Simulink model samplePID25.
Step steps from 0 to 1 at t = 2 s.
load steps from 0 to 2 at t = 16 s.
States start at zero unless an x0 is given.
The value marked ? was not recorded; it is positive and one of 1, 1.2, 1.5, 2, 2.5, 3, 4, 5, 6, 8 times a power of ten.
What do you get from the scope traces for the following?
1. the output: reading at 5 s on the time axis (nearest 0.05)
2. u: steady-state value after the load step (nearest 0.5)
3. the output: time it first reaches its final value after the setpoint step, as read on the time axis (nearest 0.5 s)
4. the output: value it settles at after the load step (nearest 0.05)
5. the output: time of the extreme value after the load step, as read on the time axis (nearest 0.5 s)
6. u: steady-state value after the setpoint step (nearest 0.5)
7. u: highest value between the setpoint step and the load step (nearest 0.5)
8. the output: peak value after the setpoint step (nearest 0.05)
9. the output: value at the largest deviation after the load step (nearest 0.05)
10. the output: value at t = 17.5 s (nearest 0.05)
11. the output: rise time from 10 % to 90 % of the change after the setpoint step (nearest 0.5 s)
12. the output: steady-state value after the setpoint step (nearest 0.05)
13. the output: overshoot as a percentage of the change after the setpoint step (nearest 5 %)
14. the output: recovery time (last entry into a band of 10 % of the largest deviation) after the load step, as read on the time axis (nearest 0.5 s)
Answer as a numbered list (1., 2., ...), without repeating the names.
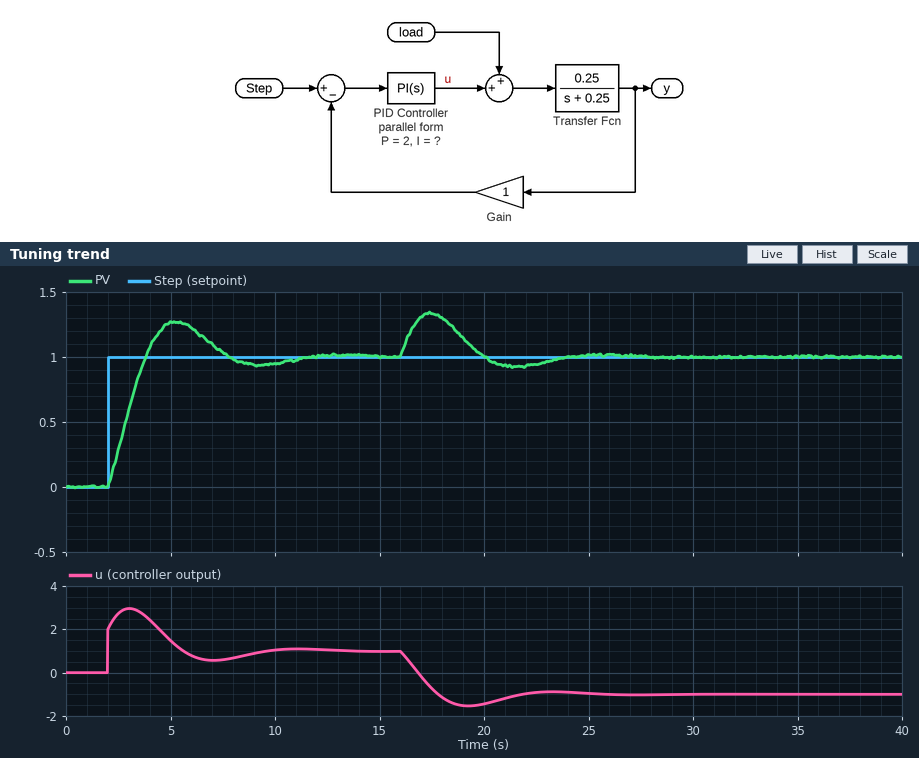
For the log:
1. 1.25
2. -1.0
3. 4.0 s
4. 1.00
5. 17.5 s
6. 1.0
7. 3.0
8. 1.25
9. 1.35
10. 1.35
11. 1.5 s
12. 1.00
13. 25 %
14. 23.0 s
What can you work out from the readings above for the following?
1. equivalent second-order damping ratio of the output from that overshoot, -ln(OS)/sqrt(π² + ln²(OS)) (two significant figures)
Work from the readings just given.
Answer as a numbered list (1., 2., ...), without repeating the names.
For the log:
1. 0.40
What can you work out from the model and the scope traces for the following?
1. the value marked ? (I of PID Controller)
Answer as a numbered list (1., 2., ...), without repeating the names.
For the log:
1. 3
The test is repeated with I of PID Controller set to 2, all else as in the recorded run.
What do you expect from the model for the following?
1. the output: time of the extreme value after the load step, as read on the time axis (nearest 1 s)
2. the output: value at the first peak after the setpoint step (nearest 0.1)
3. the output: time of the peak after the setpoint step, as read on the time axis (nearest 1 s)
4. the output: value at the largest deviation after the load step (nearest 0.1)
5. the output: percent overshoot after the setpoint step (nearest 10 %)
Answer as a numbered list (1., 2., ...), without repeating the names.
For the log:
1. 18 s
2. 1.2
3. 6 s
4. 1.4
5. 20 %
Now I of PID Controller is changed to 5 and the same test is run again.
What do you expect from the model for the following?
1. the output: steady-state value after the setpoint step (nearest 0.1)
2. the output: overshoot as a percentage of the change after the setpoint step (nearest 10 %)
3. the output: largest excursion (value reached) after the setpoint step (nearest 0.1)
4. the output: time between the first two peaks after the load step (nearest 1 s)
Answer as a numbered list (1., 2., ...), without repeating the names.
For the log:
1. 1.0
2. 40 %
3. 1.4
4. 6 s
